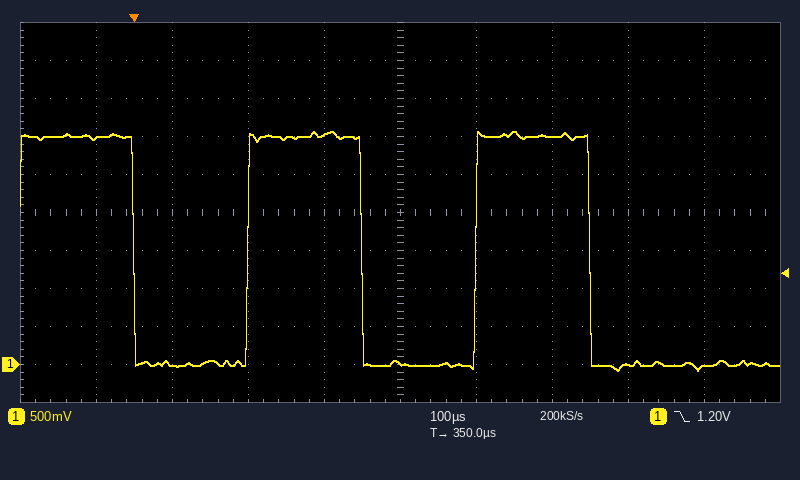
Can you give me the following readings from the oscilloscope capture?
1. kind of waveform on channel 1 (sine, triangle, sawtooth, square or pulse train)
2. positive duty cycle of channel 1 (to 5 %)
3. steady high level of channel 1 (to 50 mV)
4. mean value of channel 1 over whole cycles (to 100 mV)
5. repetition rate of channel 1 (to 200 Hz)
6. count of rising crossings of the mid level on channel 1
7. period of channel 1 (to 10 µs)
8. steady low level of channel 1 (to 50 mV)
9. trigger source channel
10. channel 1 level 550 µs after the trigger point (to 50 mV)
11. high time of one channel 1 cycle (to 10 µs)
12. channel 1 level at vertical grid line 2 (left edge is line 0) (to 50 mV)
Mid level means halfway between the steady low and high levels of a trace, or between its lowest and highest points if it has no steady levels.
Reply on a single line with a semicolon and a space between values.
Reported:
square; 50 %; 3.00 V; 1.5 V; 3.4 kHz; 2; 300 µs; 0 mV; channel 1; 3.00 V; 150 µs; 0 mV
